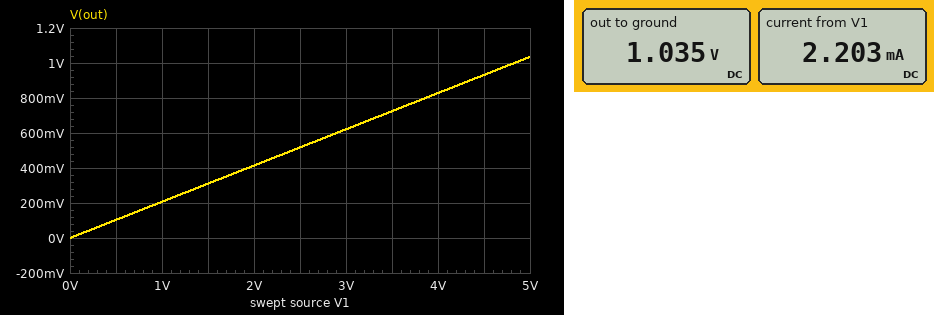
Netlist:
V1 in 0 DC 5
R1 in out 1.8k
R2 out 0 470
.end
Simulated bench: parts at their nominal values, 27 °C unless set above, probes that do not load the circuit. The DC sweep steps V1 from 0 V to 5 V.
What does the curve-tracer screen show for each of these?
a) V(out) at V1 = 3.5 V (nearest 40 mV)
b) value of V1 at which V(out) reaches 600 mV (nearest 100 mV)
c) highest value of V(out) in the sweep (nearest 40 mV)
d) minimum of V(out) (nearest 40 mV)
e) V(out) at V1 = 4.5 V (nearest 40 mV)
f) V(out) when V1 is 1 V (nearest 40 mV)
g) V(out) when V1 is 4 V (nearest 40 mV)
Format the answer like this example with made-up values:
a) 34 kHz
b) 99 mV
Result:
a) 720 mV
b) 2.9 V
c) 1.04 V
d) 0 V
e) 920 mV
f) 200 mV
g) 840 mV
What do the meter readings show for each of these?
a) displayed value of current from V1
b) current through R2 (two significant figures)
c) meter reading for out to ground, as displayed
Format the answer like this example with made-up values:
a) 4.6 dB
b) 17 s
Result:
a) 2.203 mA
b) 2.2 mA
c) 1.035 V
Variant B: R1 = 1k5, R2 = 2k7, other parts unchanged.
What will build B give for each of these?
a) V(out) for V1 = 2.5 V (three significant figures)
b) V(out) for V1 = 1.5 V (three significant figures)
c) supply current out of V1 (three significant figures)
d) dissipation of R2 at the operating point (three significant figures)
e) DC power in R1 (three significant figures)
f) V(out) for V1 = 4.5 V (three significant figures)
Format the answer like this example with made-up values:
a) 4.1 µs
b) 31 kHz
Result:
a) 1.61 V
b) 964 mV
c) 1.19 mA
d) 3.83 mW
e) 2.13 mW
f) 2.89 V
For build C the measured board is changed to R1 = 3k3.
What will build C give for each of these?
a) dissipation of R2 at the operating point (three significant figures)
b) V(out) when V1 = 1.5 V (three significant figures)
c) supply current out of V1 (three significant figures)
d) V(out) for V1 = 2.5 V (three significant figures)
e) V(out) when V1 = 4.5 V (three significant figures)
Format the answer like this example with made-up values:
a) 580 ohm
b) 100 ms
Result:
a) 827 µW
b) 187 mV
c) 1.33 mA
d) 312 mV
e) 561 mV
